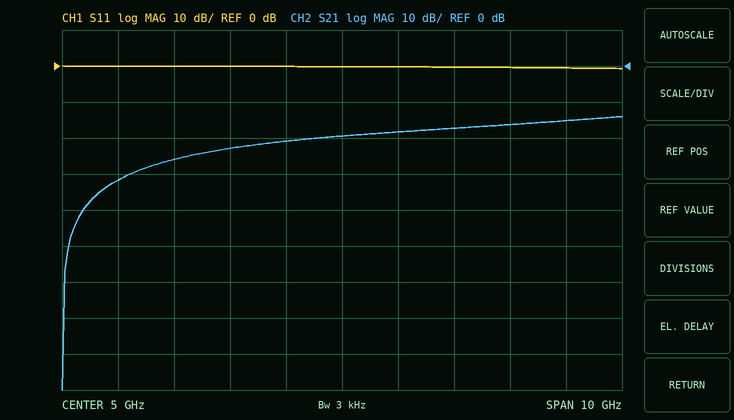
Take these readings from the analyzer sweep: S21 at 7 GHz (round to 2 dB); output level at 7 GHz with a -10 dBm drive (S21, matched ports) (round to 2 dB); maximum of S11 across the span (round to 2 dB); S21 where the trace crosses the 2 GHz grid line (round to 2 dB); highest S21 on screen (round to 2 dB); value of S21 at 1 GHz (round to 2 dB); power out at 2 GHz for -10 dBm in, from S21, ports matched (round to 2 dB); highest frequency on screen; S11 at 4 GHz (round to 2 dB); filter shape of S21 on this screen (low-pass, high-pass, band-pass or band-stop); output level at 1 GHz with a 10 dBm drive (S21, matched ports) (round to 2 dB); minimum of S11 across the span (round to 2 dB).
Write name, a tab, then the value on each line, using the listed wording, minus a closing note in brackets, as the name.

S21 at 7 GHz	-18 dB
output level at 7 GHz with a -10 dBm drive (S21, matched ports)	-28 dBm
maximum of S11 across the span	0 dB
S21 where the trace crosses the 2 GHz grid line	-26 dB
highest S21 on screen	-14 dB
value of S21 at 1 GHz	-32 dB
power out at 2 GHz for -10 dBm in, from S21, ports matched	-36 dBm
highest frequency on screen	10 GHz
S11 at 4 GHz	0 dB
filter shape of S21 on this screen	high-pass
output level at 1 GHz with a 10 dBm drive (S21, matched ports)	-22 dBm
minimum of S11 across the span	0 dB
